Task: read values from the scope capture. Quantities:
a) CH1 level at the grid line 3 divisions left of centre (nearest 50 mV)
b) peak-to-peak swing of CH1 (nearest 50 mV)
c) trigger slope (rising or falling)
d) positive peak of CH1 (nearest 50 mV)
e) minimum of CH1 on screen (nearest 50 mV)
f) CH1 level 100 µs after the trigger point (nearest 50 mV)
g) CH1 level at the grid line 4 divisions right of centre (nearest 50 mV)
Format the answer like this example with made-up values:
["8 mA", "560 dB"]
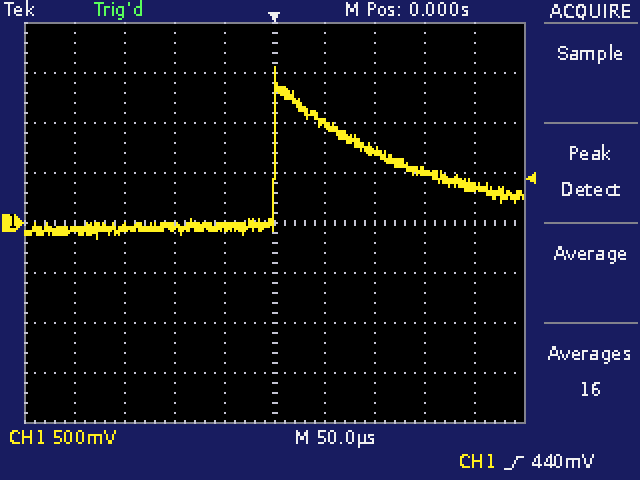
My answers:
["-50 mV", "1.70 V", "rising", "1.55 V", "-150 mV", "700 mV", "350 mV"]
